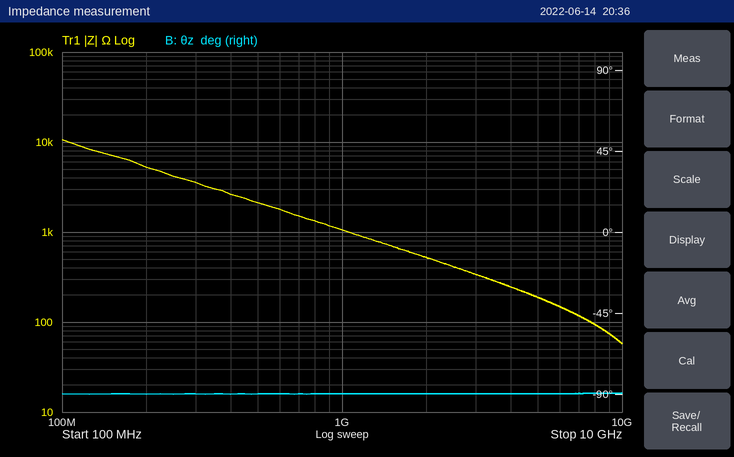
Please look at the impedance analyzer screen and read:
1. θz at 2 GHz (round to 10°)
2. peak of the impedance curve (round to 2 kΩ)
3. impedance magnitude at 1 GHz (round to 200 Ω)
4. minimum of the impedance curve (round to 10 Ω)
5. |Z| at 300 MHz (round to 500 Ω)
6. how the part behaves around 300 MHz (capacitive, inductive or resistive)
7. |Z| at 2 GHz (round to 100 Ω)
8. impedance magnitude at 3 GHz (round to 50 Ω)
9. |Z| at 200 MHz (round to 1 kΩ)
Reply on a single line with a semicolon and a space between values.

-90°; 10 kΩ; 1.0 kΩ; 60 Ω; 3.5 kΩ; capacitive; 500 Ω; 350 Ω; 5 kΩ
